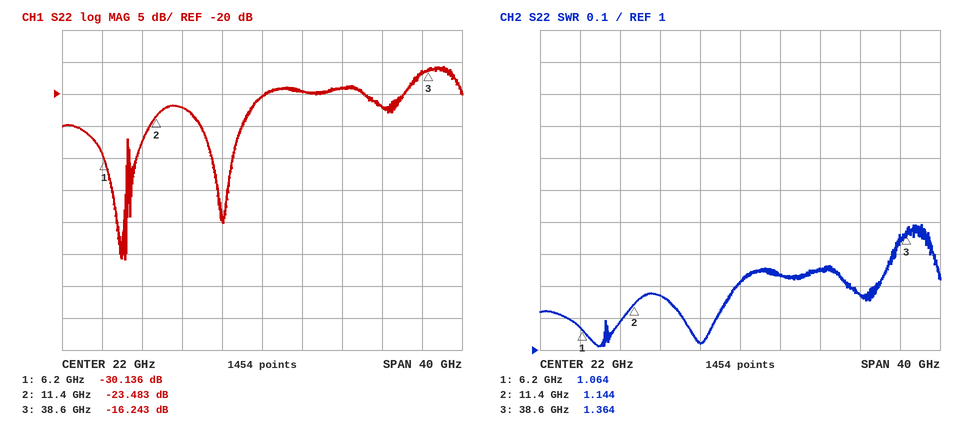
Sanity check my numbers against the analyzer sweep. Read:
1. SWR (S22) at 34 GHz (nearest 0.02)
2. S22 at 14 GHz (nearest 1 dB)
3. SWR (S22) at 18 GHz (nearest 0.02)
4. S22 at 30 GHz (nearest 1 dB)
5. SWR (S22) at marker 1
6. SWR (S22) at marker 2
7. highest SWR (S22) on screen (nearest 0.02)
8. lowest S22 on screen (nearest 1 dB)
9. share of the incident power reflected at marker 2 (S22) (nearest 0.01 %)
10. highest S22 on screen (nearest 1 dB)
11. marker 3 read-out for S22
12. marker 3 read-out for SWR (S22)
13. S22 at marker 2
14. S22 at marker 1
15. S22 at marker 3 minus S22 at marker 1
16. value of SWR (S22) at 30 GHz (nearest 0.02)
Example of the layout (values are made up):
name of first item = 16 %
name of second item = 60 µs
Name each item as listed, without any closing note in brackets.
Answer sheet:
SWR (S22) at 34 GHz = 1.18
S22 at 14 GHz = -22 dB
SWR (S22) at 18 GHz = 1.02
S22 at 30 GHz = -19 dB
SWR (S22) at marker 1 = 1.064
SWR (S22) at marker 2 = 1.144
highest SWR (S22) on screen = 1.40
lowest S22 on screen = -46 dB
share of the incident power reflected at marker 2 (S22) = 0.45 %
highest S22 on screen = -16 dB
marker 3 read-out for S22 = -16.243 dB
marker 3 read-out for SWR = 1.364
S22 at marker 2 = -23.483 dB
S22 at marker 1 = -30.136 dB
S22 at marker 3 minus S22 at marker 1 = 13.893 dB
value of SWR (S22) at 30 GHz = 1.26
